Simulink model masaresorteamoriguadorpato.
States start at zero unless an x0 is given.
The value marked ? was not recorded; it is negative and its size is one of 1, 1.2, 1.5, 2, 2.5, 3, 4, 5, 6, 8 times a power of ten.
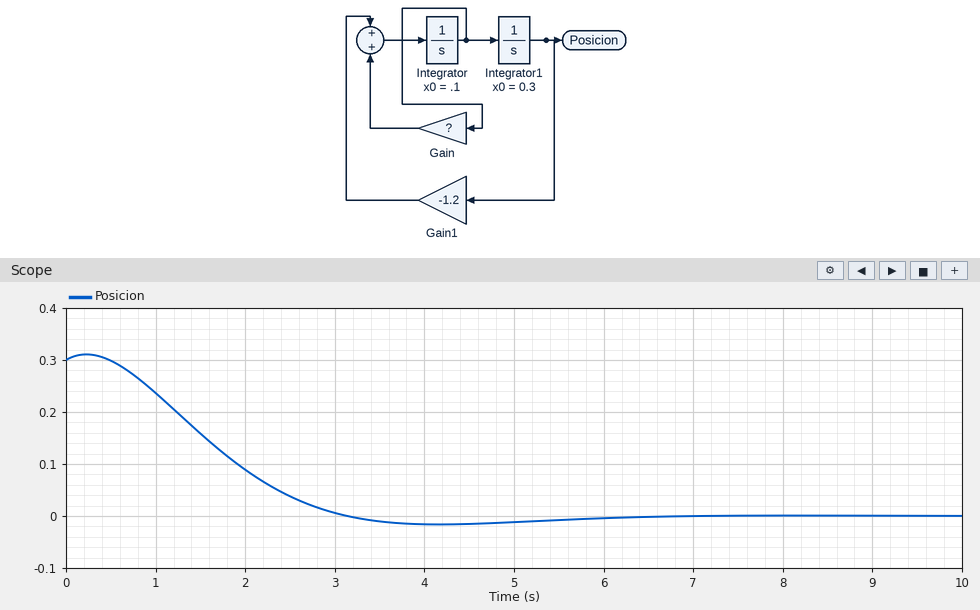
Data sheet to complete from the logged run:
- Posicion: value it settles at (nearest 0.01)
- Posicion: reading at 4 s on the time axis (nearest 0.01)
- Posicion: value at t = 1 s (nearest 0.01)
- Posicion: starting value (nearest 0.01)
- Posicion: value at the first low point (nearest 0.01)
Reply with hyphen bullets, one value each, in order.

- 0.00
- -0.02
- 0.24
- 0.30
- -0.02
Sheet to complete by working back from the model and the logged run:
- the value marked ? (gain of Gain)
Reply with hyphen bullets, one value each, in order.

- -1.5
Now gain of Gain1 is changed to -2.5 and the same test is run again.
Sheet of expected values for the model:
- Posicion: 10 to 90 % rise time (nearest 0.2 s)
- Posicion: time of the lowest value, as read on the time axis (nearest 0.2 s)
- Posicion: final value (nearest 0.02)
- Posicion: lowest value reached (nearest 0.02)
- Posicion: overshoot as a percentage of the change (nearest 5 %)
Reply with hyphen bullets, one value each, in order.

- 1.0 s
- 2.4 s
- 0.00
- -0.06
- 20 %
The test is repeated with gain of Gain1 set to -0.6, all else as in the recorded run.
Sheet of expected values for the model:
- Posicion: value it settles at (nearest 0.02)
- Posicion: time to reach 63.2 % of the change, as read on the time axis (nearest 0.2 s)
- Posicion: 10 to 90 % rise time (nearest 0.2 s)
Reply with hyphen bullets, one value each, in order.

- 0.00
- 3.2 s
- 4.0 s
